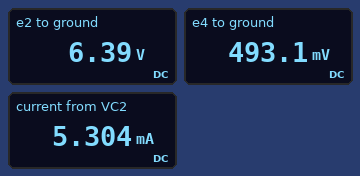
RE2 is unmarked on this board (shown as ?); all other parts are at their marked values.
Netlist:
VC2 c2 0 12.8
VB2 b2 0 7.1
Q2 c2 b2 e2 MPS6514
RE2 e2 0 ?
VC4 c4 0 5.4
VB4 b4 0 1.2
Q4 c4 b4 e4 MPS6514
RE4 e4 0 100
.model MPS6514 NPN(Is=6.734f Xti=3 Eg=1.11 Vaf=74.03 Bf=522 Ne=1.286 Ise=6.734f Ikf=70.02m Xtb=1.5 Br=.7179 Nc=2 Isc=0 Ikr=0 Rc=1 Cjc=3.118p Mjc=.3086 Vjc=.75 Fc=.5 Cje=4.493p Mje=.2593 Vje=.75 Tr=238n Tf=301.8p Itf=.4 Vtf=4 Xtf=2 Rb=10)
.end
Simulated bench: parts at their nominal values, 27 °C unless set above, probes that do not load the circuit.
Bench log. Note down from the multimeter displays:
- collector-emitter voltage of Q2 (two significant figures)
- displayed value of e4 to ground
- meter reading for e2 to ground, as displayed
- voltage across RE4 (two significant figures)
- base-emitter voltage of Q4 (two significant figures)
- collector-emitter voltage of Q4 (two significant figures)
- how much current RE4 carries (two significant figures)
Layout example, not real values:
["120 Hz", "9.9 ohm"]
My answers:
["6.4 V", "493.1 mV", "6.39 V", "490 mV", "710 mV", "4.9 V", "4.9 mA"]
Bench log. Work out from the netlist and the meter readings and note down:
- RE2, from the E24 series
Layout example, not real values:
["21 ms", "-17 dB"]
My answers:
["1.2 kΩ"]
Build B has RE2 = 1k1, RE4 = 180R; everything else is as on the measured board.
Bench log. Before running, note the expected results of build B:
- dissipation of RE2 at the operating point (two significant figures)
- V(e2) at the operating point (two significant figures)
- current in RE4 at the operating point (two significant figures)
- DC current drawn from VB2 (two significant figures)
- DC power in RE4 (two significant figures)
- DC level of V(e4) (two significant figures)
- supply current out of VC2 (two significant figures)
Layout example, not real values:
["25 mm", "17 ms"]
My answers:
["37 mW", "6.4 V", "2.8 mA", "24 µA", "1.4 mW", "510 mV", "5.8 mA"]
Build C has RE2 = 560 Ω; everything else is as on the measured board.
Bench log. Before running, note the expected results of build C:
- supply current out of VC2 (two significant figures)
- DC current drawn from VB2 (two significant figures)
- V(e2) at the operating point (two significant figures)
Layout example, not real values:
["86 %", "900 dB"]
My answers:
["11 mA", "46 µA", "6.4 V"]
